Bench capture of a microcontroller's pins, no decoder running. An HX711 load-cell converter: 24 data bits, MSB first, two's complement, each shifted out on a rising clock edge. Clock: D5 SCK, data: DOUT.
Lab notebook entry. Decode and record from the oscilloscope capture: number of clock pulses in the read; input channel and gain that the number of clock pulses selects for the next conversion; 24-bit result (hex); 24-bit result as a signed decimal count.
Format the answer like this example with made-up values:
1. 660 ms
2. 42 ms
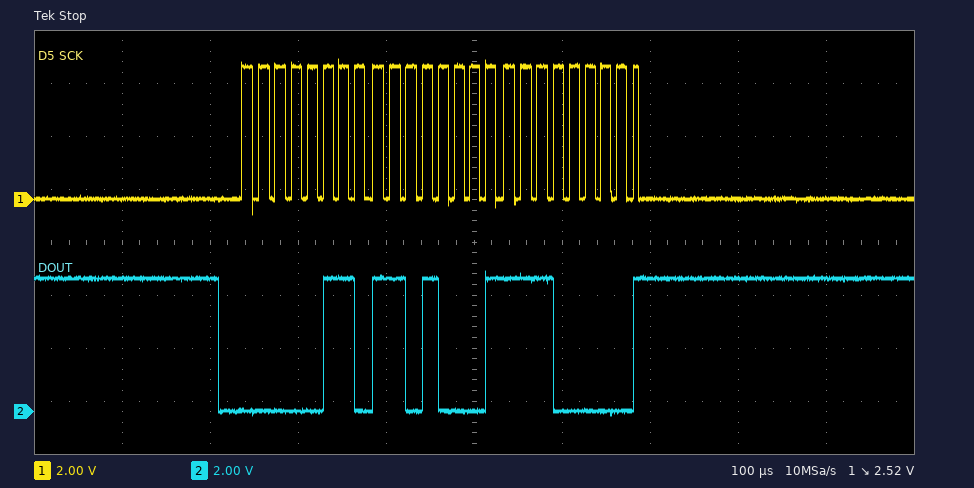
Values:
1. 25
2. channel A, gain 128
3. 0x06D1E0
4. 446944
